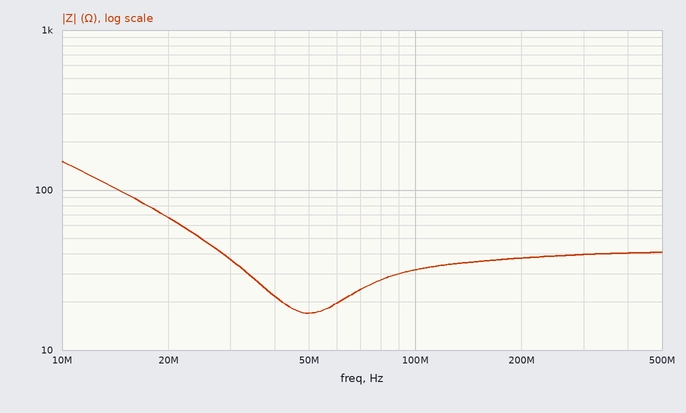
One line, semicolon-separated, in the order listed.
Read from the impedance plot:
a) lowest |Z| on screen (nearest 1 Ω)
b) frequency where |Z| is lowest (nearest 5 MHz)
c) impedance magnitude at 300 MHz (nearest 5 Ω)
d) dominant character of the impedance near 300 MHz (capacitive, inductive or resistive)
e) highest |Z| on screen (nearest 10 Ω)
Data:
17 Ω; 50 MHz; 40 Ω; resistive; 150 Ω
